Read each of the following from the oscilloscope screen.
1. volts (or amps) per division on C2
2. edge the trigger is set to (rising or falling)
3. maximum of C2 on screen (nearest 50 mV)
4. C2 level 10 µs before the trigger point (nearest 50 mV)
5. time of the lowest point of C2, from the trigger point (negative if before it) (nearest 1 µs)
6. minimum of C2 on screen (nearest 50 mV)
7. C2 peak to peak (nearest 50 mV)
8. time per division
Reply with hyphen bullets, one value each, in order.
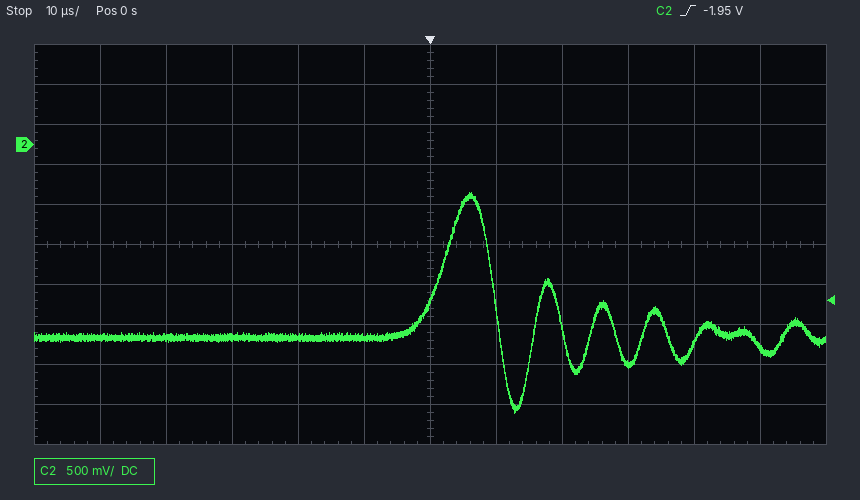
- 500 mV
- rising
- -600 mV
- -2.40 V
- +13 µs
- -3.35 V
- 2.75 V
- 10 µs
